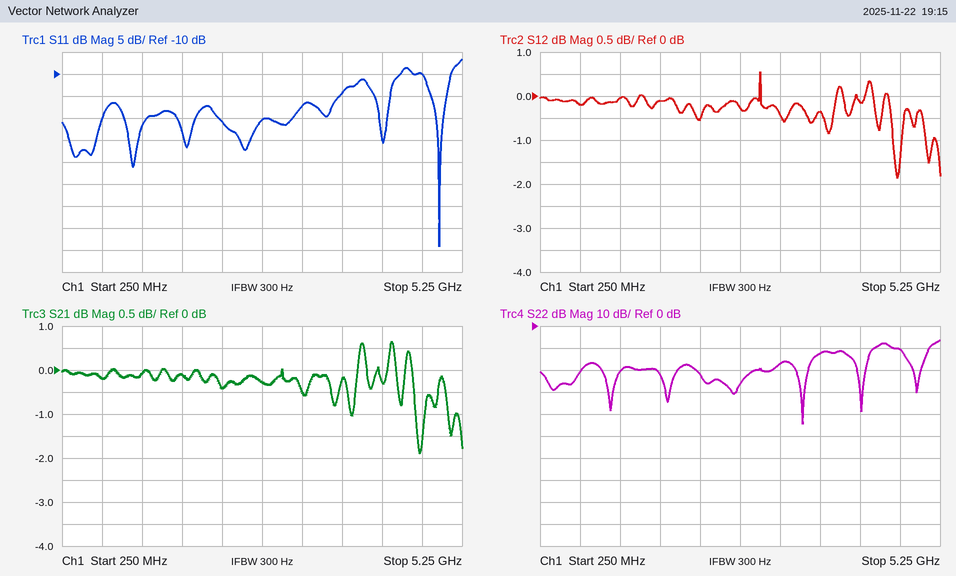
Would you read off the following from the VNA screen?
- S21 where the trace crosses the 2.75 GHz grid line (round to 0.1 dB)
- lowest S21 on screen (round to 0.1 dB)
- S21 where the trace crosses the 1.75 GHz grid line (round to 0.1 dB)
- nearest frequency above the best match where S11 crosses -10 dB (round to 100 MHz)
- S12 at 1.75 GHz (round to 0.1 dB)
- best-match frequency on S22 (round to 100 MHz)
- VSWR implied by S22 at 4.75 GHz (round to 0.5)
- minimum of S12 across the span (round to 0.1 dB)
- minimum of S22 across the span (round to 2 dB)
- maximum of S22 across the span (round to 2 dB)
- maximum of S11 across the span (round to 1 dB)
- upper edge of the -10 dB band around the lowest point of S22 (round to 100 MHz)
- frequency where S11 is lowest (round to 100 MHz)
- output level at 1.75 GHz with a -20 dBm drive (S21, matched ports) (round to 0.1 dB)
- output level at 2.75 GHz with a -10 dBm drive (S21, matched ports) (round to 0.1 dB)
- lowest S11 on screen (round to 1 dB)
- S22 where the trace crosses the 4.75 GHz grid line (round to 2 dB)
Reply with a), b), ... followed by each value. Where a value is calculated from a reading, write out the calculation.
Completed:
a) -0.3 dB
b) -1.9 dB
c) -0.1 dB
d) 5.1 GHz
e) -0.1 dB
f) 3.5 GHz
g) |Γ| = 10^(-10/20) = 0.3162; VSWR = (1 + 0.3162)/(1 − 0.3162) ≈ 1.92, so 2.0 to the nearest 0.5
h) -1.9 dB
i) -44 dB
j) -6 dB
k) -7 dB
l) 4.4 GHz
m) 5.0 GHz
n) -20 dBm + (-0.1 dB) = -20.1 dBm
o) -10 dBm + (-0.3 dB) = -10.3 dBm
p) -49 dB
q) -10 dB
